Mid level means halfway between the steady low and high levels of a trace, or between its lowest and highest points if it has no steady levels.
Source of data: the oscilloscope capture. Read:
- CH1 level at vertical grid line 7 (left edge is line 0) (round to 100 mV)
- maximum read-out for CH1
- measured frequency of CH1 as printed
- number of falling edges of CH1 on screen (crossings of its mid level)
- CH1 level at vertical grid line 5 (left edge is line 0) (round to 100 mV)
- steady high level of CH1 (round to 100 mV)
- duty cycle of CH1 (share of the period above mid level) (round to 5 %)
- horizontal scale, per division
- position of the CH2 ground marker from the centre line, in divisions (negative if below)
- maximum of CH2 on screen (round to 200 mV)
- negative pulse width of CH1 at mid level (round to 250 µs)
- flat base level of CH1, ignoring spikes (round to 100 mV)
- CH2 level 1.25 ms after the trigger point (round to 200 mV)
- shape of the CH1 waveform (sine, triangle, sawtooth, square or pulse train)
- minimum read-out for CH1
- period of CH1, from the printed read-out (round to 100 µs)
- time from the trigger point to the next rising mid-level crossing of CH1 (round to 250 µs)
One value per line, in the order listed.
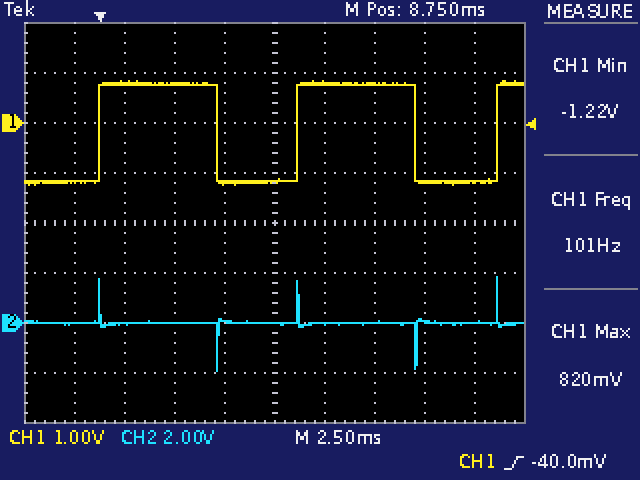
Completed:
800 mV
820 mV
101 Hz
2
-1.2 V
800 mV
60 %
2.5 ms
-2.0 div
1.8 V
4.00 ms
-1.2 V
0.0 V
pulse train
-1.22 V
9.9 ms
10.00 ms
